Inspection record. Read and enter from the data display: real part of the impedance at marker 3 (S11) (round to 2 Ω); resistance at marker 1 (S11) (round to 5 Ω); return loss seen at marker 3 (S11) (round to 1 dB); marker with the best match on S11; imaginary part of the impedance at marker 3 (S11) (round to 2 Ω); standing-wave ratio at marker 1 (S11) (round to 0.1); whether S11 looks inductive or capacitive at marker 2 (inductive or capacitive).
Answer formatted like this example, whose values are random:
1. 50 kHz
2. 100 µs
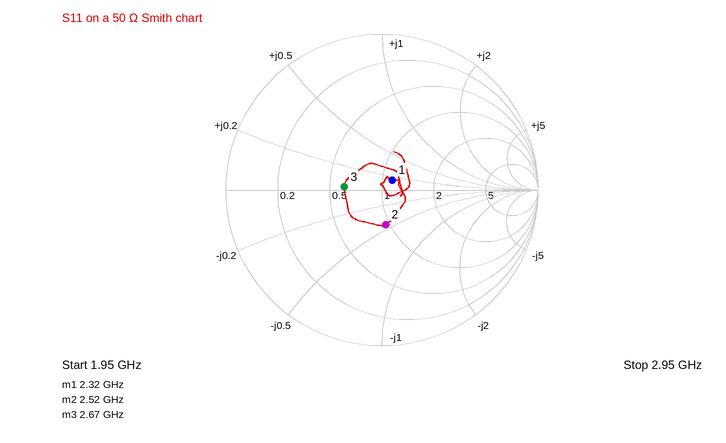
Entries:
1. 30 Ω
2. 55 Ω
3. 12 dB
4. marker 1
5. +2 Ω
6. 1.2
7. capacitive
